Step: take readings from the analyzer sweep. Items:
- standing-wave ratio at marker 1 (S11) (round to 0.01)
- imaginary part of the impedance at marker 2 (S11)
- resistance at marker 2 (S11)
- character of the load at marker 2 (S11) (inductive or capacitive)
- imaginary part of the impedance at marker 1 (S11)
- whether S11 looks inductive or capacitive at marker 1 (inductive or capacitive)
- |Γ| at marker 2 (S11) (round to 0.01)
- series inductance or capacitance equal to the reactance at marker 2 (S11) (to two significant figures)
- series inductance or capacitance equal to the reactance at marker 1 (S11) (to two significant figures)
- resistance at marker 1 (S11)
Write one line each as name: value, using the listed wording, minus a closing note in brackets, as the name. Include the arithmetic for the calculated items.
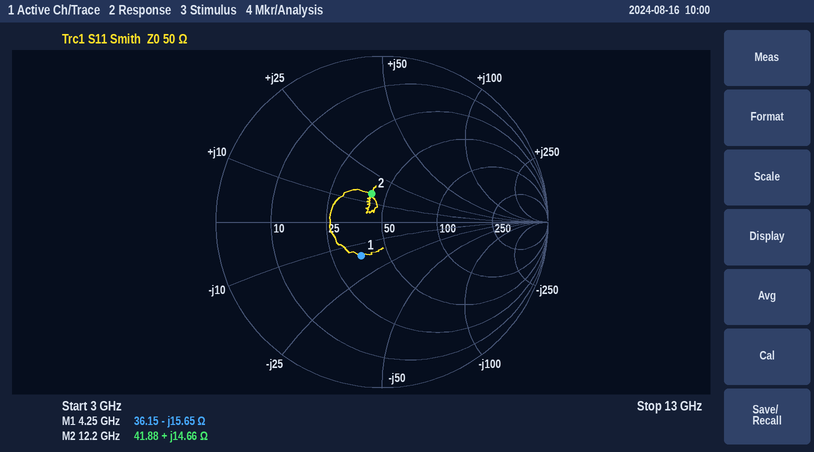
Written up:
standing-wave ratio at marker 1 (S11): 1.63
imaginary part of the impedance at marker 2: +14.66 Ω
resistance at marker 2: 41.88 Ω
character of the load at marker 2 (S11): inductive
imaginary part of the impedance at marker 1: -15.65 Ω
whether S11 looks inductive or capacitive at marker 1: capacitive
|Γ| at marker 2 (S11): 0.18
series inductance or capacitance equal to the reactance at marker 2 (S11): L = 14.66 Ω/(2π × 12.2 GHz) ≈ 191 pH, so 190 pH to two significant figures
series inductance or capacitance equal to the reactance at marker 1 (S11): C = 1/(2π × 4.25 GHz × 15.65 Ω) ≈ 2.4 pF
resistance at marker 1: 36.15 Ω
